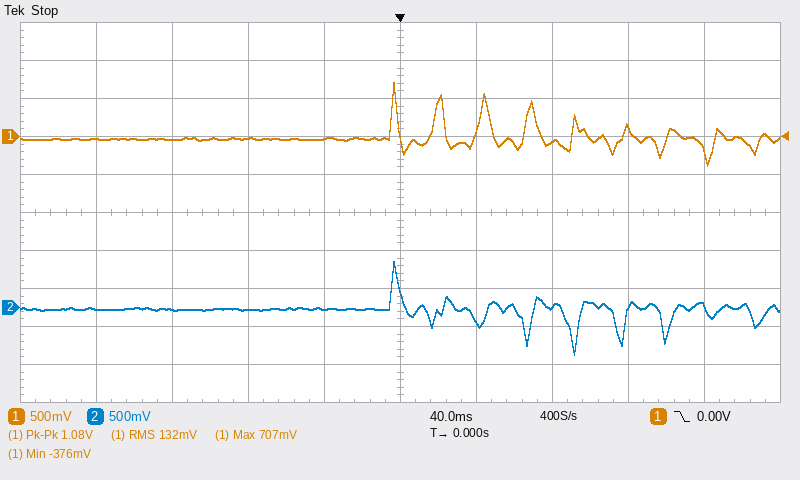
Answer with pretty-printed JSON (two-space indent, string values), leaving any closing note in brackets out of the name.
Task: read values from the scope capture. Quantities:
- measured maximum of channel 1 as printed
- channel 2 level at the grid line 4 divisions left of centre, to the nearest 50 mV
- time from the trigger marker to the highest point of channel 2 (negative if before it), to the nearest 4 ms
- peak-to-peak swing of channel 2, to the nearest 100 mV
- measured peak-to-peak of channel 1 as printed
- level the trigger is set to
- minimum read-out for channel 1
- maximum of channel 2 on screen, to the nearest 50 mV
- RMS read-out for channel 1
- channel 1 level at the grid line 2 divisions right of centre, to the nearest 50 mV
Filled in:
{
  "measured maximum of channel 1 as printed": "707 mV",
  "channel 2 level at the grid line 4 divisions left of centre, to the nearest 50 mV": "0 mV",
  "time from the trigger marker to the highest point of channel 2 (negative if before it), to the nearest 4 ms": "-4 ms",
  "peak-to-peak swing of channel 2, to the nearest 100 mV": "1.20 V",
  "measured peak-to-peak of channel 1 as printed": "1.08 V",
  "level the trigger is set to": "0.00 V",
  "minimum read-out for channel 1": "-376 mV",
  "maximum of channel 2 on screen, to the nearest 50 mV": "600 mV",
  "RMS read-out for channel 1": "132 mV",
  "channel 1 level at the grid line 2 divisions right of centre, to the nearest 50 mV": "-50 mV"
}
